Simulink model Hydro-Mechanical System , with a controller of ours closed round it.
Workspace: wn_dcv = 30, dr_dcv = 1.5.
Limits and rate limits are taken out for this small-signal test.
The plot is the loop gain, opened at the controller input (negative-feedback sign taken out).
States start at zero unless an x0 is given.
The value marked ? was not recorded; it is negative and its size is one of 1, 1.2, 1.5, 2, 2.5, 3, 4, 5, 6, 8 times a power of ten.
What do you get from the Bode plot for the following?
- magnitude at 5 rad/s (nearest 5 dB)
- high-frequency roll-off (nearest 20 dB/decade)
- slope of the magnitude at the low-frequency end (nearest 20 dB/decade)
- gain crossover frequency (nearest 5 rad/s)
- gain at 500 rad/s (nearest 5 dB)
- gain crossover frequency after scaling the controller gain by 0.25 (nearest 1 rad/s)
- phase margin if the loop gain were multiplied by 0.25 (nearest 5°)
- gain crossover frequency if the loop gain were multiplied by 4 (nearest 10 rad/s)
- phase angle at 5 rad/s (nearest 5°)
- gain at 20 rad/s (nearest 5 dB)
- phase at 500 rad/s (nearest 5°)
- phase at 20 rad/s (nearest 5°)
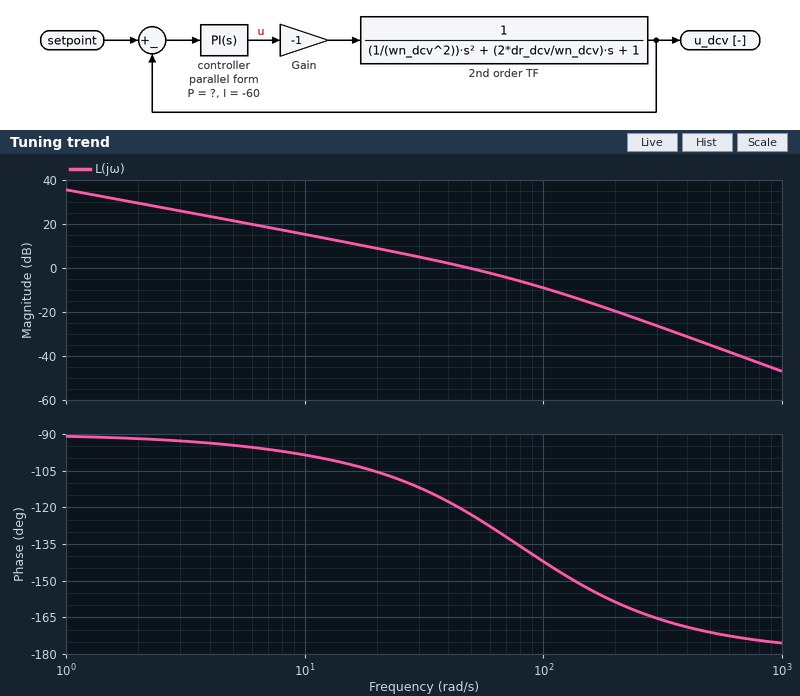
20 dB
-40 dB/decade
-20 dB/decade
50 rad/s
-35 dB
14 rad/s
80°
120 rad/s
-95°
10 dB
-170°
-105°
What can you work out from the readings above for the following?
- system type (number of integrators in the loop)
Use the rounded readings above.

1
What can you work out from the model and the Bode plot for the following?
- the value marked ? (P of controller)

-5
